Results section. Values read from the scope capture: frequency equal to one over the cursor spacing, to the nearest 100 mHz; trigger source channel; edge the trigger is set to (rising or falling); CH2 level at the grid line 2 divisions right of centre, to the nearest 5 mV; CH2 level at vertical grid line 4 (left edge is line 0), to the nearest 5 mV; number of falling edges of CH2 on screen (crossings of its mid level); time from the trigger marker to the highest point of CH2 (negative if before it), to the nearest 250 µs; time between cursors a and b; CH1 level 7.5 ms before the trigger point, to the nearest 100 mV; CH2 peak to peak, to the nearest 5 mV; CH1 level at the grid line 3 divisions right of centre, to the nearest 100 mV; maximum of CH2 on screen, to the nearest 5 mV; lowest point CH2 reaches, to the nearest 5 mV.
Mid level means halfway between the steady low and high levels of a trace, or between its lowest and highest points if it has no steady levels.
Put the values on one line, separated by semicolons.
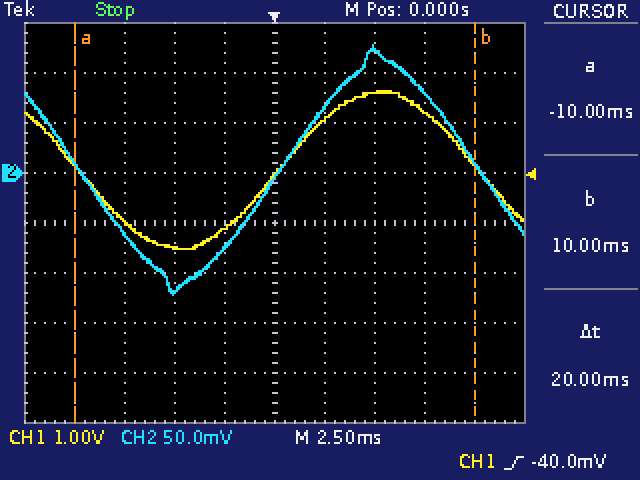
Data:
50.0 Hz; CH1; rising; 125 mV; -75 mV; 2; +5.00 ms; 20 ms; -1.0 V; 250 mV; 1.2 V; 130 mV; -120 mV
